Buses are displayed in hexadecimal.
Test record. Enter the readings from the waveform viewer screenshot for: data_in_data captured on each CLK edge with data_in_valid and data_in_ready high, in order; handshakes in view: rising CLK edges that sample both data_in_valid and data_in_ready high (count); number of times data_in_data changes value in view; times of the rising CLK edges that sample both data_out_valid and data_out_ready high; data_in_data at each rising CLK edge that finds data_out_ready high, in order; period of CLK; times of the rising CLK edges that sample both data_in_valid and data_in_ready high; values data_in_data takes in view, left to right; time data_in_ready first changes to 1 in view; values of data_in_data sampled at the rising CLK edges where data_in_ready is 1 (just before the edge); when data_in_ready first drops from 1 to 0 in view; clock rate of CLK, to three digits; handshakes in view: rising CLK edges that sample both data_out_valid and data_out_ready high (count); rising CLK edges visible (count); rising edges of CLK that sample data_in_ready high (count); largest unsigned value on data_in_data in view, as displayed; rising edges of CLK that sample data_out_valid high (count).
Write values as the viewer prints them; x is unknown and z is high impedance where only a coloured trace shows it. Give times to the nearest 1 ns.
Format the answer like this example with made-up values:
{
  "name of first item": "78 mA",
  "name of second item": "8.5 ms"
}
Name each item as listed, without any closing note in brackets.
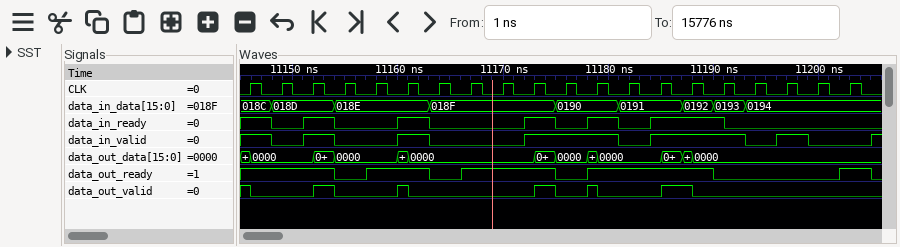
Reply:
{
  "data_in_data captured on each CLK edge with data_in_valid and data_in_ready high, in order": "018C, 018D, 018E, 018F, 0190, 0191, 0192, 0193",
  "handshakes in view: rising CLK edges that sample both data_in_valid and data_in_ready high": "8",
  "number of times data_in_data changes value in view": "8",
  "times of the rising CLK edges that sample both data_out_valid and data_out_ready high": "11146 ns, 11161 ns, 11179 ns, 11188 ns",
  "data_in_data at each rising CLK edge that finds data_out_ready high, in order": "018C, 018D, 018D, 018E, 018E, 018F, 018F, 018F, 0190, 0191, 0191, 0192, 0194",
  "period of CLK": "3 ns",
  "times of the rising CLK edges that sample both data_in_valid and data_in_ready high": "11146 ns, 11152 ns, 11161 ns, 11173 ns, 11179 ns, 11185 ns, 11188 ns, 11191 ns",
  "values data_in_data takes in view, left to right": "018C, 018D, 018E, 018F, 0190, 0191, 0192, 0193, 0194",
  "time data_in_ready first changes to 1 in view": "11151 ns",
  "values of data_in_data sampled at the rising CLK edges where data_in_ready is 1": "018C, 018D, 018E, 018F, 0190, 0191, 0192, 0193",
  "when data_in_ready first drops from 1 to 0 in view": "11148 ns",
  "clock rate of CLK, to three digits": "333 MHz",
  "handshakes in view: rising CLK edges that sample both data_out_valid and data_out_ready high": "4",
  "rising CLK edges visible": "20",
  "rising edges of CLK that sample data_in_ready high": "8",
  "largest unsigned value on data_in_data in view, as displayed": "0194",
  "rising edges of CLK that sample data_out_valid high": "4"
}
